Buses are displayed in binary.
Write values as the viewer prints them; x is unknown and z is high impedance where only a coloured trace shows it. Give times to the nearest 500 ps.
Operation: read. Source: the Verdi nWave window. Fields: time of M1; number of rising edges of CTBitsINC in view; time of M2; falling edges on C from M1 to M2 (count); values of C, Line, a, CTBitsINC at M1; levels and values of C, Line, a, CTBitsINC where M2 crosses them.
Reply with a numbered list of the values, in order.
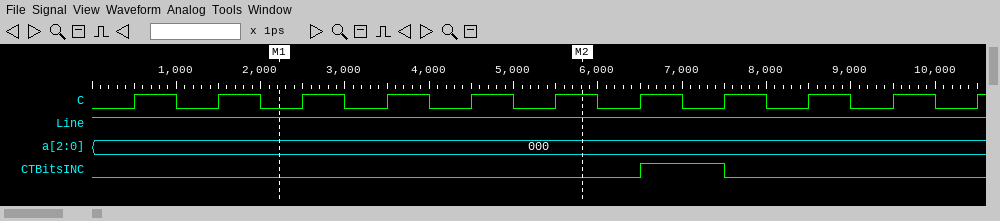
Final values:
1. 2000 ps
2. 1
3. 6000 ps
4. 3
5. C=0, Line=1, a=000, CTBitsINC=0
6. C=1, Line=1, a=000, CTBitsINC=0
